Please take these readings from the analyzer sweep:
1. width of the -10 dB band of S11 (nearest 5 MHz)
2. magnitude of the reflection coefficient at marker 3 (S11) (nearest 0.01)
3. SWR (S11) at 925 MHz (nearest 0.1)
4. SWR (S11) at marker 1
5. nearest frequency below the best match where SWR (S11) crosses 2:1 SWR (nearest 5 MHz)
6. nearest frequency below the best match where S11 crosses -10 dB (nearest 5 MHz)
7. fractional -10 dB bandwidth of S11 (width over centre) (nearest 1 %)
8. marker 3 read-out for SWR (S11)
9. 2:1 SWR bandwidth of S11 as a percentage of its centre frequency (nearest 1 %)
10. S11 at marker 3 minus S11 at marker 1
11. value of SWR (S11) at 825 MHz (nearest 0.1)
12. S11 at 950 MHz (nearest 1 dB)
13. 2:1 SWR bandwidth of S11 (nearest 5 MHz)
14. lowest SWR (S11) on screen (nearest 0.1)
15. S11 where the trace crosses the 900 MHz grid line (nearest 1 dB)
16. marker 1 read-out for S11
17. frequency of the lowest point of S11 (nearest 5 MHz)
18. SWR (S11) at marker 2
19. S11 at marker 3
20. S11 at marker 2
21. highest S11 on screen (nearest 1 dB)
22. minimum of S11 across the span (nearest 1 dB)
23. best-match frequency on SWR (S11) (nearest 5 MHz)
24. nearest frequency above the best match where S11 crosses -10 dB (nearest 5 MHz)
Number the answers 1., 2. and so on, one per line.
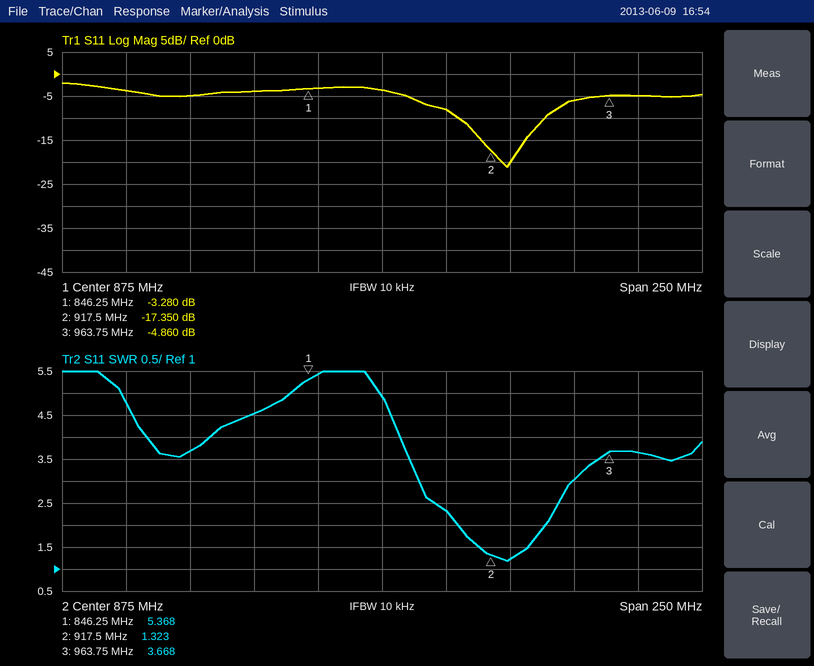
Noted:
1. 35 MHz
2. 0.57
3. 1.2
4. 5.368
5. 905 MHz
6. 905 MHz
7. 4 %
8. 3.668
9. 4 %
10. -1.580 dB
11. 4.5
12. -6 dB
13. 35 MHz
14. 1.2
15. -8 dB
16. -3.280 dB
17. 925 MHz
18. 1.323
19. -4.860 dB
20. -17.350 dB
21. -2 dB
22. -21 dB
23. 925 MHz
24. 940 MHz
